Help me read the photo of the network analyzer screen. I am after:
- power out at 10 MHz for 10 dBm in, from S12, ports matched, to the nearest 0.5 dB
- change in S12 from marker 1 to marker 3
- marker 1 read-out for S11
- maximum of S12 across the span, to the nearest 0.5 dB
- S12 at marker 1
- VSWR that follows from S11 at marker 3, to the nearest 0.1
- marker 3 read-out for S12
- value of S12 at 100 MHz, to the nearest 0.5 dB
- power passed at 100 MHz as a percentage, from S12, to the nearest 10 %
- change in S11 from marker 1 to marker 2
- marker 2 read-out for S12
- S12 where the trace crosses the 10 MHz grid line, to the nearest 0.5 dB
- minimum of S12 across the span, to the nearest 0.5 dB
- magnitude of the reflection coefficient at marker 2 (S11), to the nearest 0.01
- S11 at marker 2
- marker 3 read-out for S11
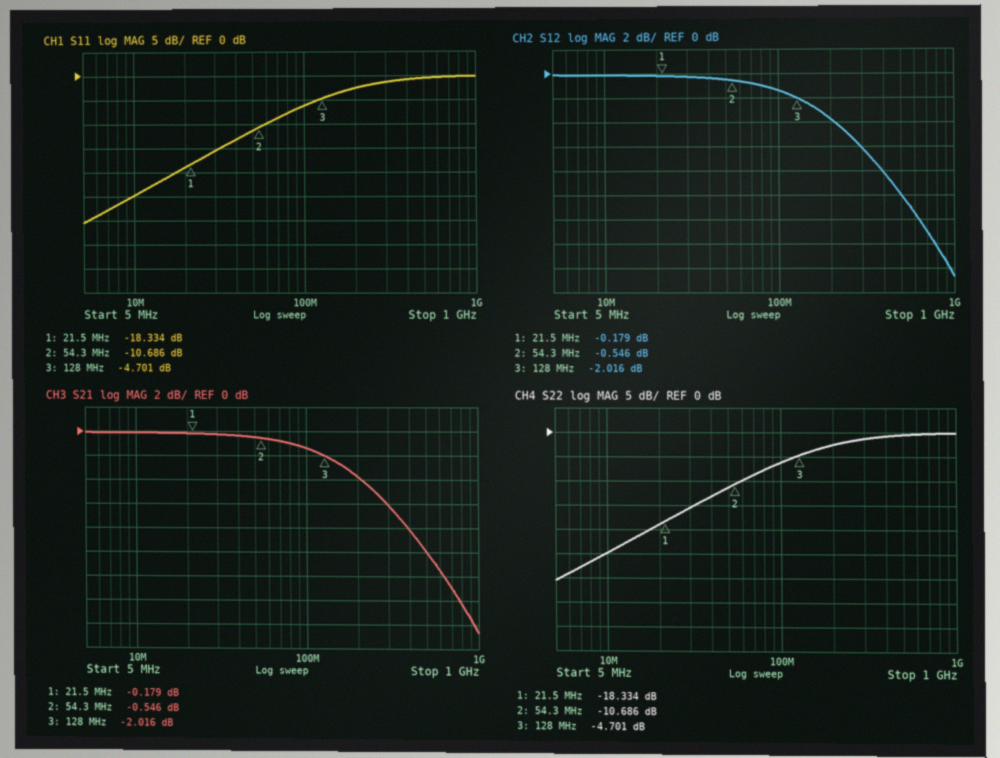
10.0 dBm
-1.837 dB
-18.334 dB
0.0 dB
-0.179 dB
3.8
-2.016 dB
-1.5 dB
70 %
7.648 dB
-0.546 dB
0.0 dB
-16.5 dB
0.29
-10.686 dB
-4.701 dB
